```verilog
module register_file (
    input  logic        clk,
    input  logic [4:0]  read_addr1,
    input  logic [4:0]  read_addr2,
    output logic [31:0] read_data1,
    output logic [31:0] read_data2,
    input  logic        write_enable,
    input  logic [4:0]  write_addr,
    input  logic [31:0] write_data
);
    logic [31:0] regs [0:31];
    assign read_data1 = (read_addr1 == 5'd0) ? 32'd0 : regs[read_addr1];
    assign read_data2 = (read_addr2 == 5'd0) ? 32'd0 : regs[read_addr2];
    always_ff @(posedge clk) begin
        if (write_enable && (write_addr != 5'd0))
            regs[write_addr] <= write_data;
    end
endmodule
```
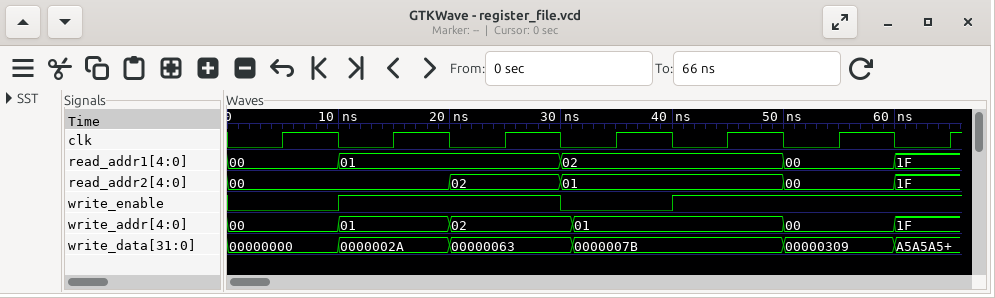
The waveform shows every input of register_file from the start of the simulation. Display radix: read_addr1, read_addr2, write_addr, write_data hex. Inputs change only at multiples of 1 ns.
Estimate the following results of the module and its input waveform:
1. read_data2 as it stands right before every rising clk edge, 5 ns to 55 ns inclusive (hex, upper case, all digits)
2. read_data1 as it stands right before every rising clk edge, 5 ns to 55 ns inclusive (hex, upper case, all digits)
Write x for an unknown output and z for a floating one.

00000000, 00000000, x, 0000002A, 0000002A, 00000000
00000000, x, 0000002A, 00000063, 00000063, 00000000
